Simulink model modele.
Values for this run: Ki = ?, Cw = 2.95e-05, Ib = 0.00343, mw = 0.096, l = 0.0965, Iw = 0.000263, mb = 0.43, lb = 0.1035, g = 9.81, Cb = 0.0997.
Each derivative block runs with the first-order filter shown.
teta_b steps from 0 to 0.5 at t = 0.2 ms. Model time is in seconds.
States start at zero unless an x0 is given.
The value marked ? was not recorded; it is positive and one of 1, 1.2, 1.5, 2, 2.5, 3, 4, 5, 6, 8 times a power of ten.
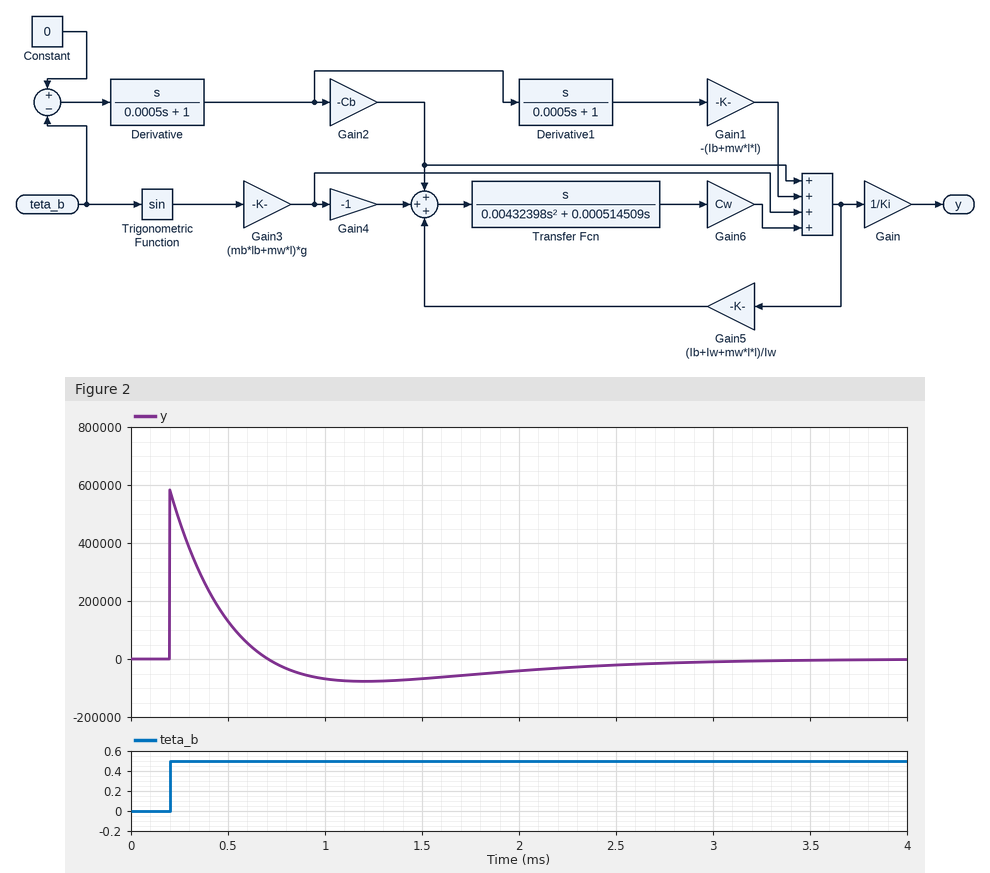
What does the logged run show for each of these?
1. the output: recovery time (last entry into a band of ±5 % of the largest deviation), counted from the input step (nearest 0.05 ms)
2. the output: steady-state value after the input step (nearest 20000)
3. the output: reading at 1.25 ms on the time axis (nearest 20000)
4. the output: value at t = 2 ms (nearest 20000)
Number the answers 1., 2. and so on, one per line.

1. 2.05 ms
2. 0
3. -80000
4. -40000
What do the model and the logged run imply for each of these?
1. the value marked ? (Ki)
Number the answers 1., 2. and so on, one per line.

1. 0.015
